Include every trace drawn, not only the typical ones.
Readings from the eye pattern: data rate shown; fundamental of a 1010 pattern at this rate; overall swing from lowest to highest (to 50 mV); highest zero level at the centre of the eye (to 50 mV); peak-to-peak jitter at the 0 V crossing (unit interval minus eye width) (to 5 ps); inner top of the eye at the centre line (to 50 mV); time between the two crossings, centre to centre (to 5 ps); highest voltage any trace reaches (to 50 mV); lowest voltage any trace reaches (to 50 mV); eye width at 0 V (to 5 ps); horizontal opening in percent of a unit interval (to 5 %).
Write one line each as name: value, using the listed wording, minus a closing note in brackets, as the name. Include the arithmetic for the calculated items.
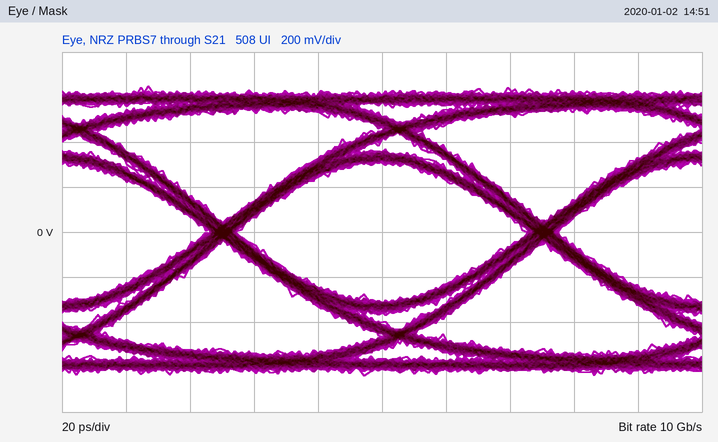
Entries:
data rate shown: 10 Gb/s
fundamental of a 1010 pattern at this rate: 5 GHz
overall swing from lowest to highest: 1.30 V
highest zero level at the centre of the eye: -300 mV
peak-to-peak jitter at the 0 V crossing (unit interval minus eye width): 10 ps
inner top of the eye at the centre line: 300 mV
time between the two crossings, centre to centre: 100 ps
highest voltage any trace reaches: 650 mV
lowest voltage any trace reaches: -650 mV
eye width at 0 V: 90 ps
horizontal opening in percent of a unit interval: 90 ps / 100 ps ≈ 90 %
